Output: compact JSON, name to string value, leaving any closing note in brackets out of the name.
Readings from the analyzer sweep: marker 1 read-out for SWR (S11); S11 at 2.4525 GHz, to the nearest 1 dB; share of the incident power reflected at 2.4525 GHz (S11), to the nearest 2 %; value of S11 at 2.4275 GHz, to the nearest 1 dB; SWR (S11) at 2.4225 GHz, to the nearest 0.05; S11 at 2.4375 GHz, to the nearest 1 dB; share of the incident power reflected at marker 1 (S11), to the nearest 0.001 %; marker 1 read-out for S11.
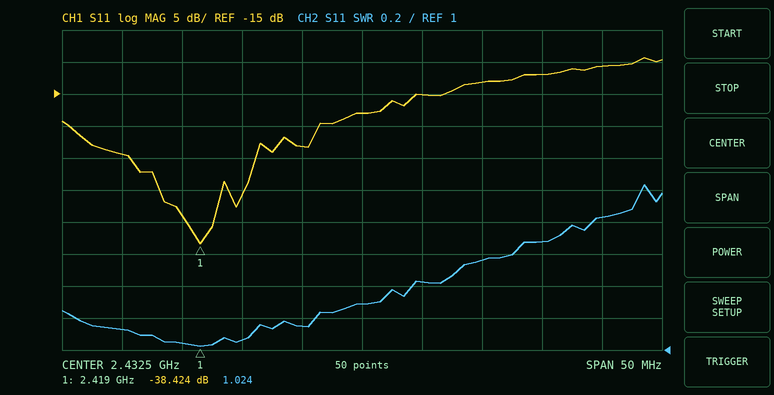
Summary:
{"marker 1 read-out for SWR": "1.024", "S11 at 2.4525 GHz, to the nearest 1 dB": "-11 dB", "share of the incident power reflected at 2.4525 GHz (S11), to the nearest 2 %": "8 %", "value of S11 at 2.4275 GHz, to the nearest 1 dB": "-23 dB", "SWR (S11) at 2.4225 GHz, to the nearest 0.05": "1.05", "S11 at 2.4375 GHz, to the nearest 1 dB": "-15 dB", "share of the incident power reflected at marker 1 (S11), to the nearest 0.001 %": "0.014 %", "marker 1 read-out for S11": "-38.424 dB"}
